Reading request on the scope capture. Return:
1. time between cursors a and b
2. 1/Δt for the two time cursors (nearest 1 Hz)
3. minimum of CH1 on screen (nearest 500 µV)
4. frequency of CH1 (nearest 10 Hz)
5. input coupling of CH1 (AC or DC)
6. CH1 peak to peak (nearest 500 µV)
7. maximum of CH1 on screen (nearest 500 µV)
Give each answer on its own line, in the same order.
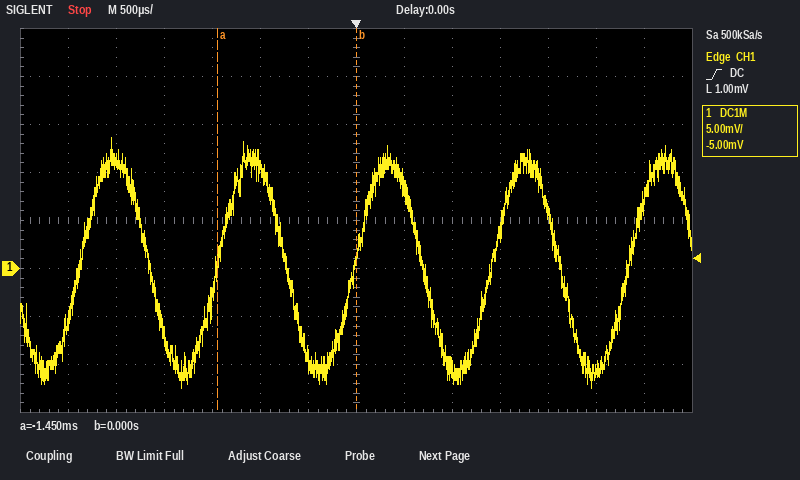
1.45 ms
690 Hz
-12.5 mV
700 Hz
DC
26.0 mV
13.5 mV
